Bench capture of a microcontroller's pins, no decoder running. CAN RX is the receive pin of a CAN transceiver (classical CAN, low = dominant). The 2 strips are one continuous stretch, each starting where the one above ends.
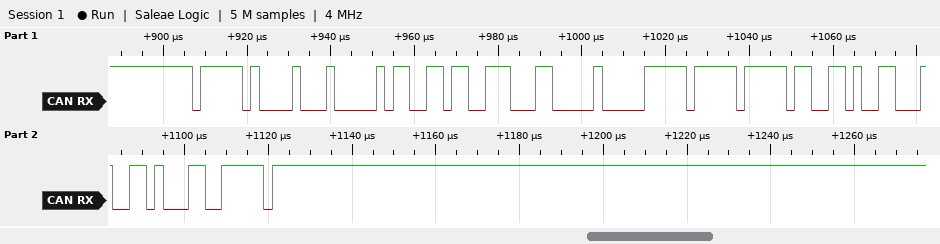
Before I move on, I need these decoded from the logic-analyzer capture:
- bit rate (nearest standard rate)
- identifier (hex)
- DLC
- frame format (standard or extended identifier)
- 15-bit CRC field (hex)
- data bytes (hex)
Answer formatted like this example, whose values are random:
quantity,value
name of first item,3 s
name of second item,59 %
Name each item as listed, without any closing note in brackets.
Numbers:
quantity,value
bit rate,500 kbit/s
identifier,0x7E1
DLC,8
frame format,standard
15-bit CRC field,0x68CF
data bytes,19 B3 8C 00 FF FF 34 C4
